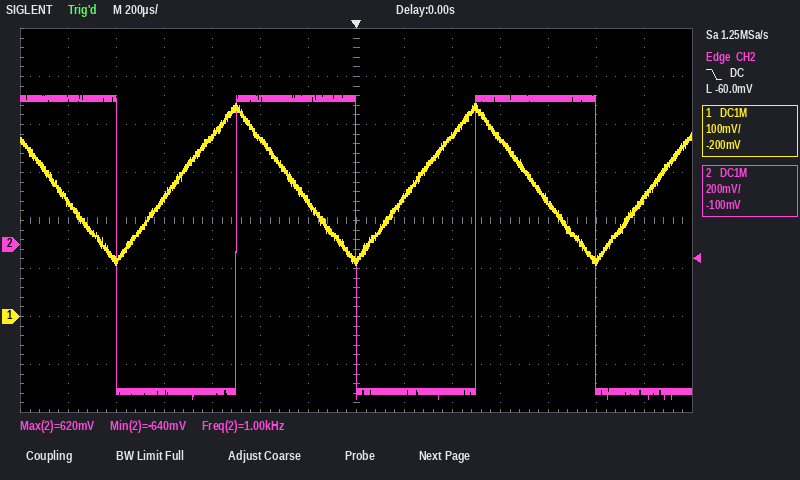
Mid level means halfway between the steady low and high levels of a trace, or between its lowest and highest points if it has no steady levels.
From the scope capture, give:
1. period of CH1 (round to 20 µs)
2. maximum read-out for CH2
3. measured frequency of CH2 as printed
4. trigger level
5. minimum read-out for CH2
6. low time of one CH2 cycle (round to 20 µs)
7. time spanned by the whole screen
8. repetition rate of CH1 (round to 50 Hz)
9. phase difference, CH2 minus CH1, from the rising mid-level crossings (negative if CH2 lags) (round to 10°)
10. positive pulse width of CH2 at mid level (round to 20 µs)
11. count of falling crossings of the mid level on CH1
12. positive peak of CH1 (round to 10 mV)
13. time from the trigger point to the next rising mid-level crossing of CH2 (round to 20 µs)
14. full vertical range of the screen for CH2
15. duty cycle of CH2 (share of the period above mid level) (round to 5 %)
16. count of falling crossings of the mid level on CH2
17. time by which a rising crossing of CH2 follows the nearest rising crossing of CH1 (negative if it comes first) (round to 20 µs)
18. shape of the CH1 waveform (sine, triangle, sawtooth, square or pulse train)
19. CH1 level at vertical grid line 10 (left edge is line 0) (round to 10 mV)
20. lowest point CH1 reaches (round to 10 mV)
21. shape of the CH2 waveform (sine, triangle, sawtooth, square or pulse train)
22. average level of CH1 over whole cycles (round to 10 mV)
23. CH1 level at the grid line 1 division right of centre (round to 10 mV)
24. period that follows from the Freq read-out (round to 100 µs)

1.00 ms
620 mV
1.00 kHz
-60.0 mV
-640 mV
500 µs
2.8 ms
1.00 kHz
-90°
500 µs
3
440 mV
500 µs
1.6 V
50 %
3
+260 µs
triangle
370 mV
110 mV
square
280 mV
250 mV
1.0 ms
